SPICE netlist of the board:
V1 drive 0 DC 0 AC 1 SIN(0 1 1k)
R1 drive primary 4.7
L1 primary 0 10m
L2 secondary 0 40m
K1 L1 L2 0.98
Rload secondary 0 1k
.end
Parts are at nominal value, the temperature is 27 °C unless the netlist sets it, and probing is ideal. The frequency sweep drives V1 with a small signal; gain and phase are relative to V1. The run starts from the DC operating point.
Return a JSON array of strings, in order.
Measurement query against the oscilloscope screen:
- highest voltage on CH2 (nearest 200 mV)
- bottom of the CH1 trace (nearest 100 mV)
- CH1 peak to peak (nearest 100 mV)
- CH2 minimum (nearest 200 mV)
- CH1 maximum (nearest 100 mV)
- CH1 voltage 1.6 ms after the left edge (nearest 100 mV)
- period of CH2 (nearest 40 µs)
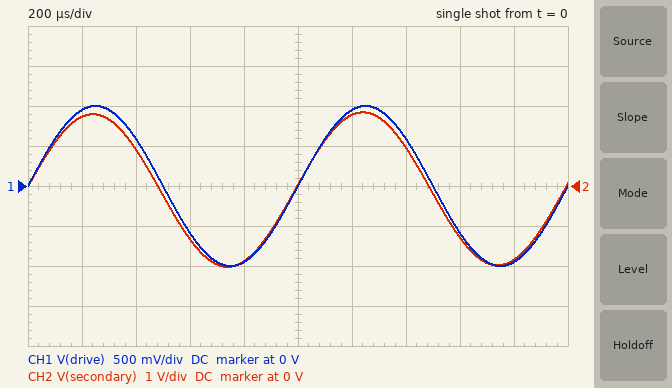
["1.8 V", "-1.0 V", "2.0 V", "-2.0 V", "1.0 V", "-600 mV", "1.00 ms"]
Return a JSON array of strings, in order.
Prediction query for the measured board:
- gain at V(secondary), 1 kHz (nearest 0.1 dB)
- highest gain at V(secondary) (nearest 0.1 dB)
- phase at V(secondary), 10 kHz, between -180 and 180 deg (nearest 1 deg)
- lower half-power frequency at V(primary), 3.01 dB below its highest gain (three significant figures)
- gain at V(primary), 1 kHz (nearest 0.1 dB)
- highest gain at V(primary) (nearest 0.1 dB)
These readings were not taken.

["5.7 dB", "5.7 dB", "-5 deg", "76.2 Hz", "-0.2 dB", "0 dB"]
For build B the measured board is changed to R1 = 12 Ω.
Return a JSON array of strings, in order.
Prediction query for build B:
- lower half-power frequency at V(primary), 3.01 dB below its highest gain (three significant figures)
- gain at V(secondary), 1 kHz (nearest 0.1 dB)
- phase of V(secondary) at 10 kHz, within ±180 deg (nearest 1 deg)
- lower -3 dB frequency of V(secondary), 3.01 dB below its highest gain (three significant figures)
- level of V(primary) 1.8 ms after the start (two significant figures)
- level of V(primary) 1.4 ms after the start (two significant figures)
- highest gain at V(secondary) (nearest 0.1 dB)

["201 Hz", "5.3 dB", "-4 deg", "182 Hz", "-850 mV", "370 mV", "5.4 dB"]
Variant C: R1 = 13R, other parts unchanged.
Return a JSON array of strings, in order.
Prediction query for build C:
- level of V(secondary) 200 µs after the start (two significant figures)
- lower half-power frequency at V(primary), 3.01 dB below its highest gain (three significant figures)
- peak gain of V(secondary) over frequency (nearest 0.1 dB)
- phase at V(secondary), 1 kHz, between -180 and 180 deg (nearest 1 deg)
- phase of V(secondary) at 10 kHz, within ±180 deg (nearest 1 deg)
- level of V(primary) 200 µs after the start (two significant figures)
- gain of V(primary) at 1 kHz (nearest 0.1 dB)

["1.5 V", "218 Hz", "5.4 dB", "11 deg", "-4 deg", "790 mV", "-0.6 dB"]
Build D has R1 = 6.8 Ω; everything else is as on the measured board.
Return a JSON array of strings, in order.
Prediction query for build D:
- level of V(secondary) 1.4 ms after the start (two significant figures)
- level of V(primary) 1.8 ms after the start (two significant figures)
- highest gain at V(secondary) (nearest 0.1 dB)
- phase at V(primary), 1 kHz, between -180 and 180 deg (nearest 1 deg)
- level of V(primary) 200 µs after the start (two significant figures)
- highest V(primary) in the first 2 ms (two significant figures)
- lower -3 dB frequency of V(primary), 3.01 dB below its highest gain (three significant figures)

["890 mV", "-920 mV", "5.6 dB", "6 deg", "860 mV", "920 mV", "111 Hz"]
